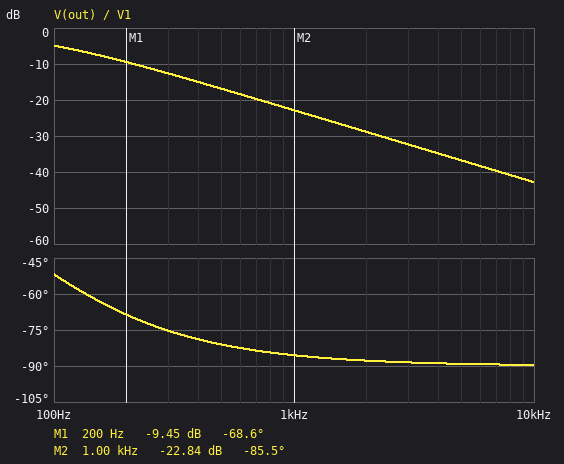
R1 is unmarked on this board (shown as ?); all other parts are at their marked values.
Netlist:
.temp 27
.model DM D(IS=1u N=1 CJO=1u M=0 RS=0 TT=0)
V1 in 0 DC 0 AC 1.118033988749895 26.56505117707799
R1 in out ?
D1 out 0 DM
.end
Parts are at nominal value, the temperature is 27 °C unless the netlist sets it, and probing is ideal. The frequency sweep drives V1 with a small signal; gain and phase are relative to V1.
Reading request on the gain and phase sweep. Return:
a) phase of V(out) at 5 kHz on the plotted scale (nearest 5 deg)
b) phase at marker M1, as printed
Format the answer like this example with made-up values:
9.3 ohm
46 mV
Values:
-90 deg
-68.6 deg
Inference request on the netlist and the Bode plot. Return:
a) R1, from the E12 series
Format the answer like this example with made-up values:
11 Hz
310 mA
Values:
2.2 kΩ
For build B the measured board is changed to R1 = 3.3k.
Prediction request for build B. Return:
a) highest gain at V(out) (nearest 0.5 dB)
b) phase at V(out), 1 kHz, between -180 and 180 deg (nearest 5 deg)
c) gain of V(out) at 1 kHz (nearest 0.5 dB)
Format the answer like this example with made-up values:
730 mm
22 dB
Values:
-1.0 dB
-85 deg
-26.5 dB
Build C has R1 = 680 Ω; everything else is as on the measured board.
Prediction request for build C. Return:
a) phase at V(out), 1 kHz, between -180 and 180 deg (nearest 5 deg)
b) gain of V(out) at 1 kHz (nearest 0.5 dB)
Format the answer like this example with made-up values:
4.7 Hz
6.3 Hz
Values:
-75 deg
-13.0 dB
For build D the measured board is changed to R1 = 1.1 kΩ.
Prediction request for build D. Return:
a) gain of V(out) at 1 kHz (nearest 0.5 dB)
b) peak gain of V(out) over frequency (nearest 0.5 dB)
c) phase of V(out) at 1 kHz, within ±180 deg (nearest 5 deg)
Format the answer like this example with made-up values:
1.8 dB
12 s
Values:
-17.0 dB
-0.5 dB
-80 deg
